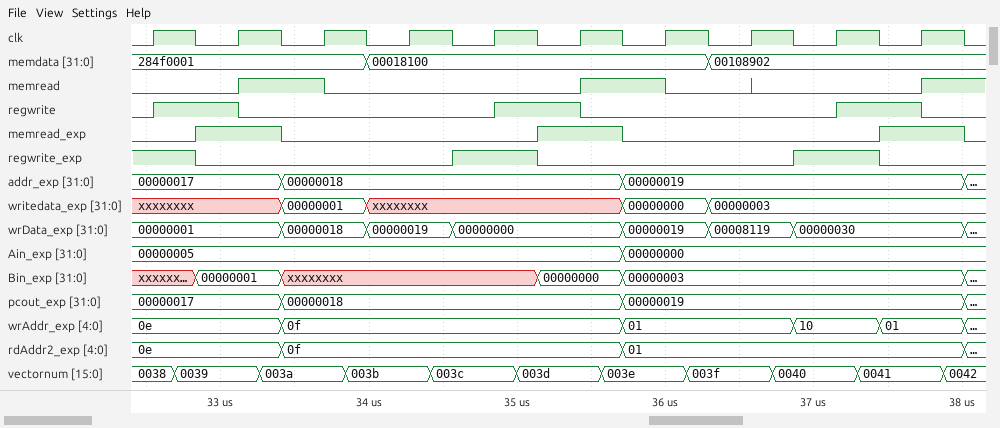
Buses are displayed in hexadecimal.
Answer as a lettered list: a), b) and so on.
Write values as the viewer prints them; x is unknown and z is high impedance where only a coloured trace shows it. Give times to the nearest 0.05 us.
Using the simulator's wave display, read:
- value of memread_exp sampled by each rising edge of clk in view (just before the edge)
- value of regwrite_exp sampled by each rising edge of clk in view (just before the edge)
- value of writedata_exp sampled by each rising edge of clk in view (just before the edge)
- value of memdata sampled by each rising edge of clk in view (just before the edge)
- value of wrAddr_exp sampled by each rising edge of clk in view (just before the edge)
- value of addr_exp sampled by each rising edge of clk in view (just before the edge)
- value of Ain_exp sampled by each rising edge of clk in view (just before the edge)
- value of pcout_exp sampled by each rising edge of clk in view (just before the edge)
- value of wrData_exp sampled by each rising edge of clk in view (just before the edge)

a) 0 1 0 0 0 1 0 0 0 1
b) 1 0 0 0 1 0 0 0 1 0
c) xxxxxxxx, xxxxxxxx, 00000001, xxxxxxxx, xxxxxxxx, xxxxxxxx, 00000000, 00000003, 00000003, 00000003
d) 284f0001, 284f0001, 284f0001, 00018100, 00018100, 00018100, 00018100, 00108902, 00108902, 00108902
e) 0e, 0e, 0f, 0f, 0f, 0f, 01, 01, 10, 01
f) 00000017, 00000017, 00000018, 00000018, 00000018, 00000018, 00000019, 00000019, 00000019, 00000019
g) 00000005, 00000005, 00000005, 00000005, 00000005, 00000005, 00000000, 00000000, 00000000, 00000000
h) 00000017, 00000017, 00000018, 00000018, 00000018, 00000018, 00000019, 00000019, 00000019, 00000019
i) 00000001, 00000001, 00000018, 00000019, 00000000, 00000000, 00000019, 00008119, 00000030, 00000030
